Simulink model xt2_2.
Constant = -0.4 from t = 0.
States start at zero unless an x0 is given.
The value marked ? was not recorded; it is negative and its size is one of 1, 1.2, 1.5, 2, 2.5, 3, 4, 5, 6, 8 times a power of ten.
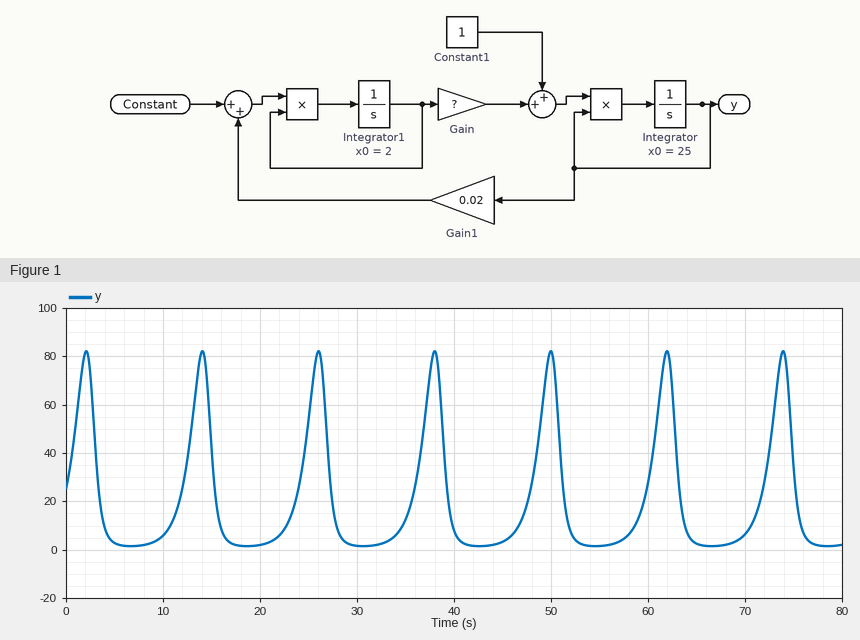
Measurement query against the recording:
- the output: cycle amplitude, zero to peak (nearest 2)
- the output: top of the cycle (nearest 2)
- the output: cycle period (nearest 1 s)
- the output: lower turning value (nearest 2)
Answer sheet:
40
82
12 s
2
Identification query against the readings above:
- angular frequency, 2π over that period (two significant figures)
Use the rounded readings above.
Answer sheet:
0.52 rad/s
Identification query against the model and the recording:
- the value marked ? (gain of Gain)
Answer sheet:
-0.12
